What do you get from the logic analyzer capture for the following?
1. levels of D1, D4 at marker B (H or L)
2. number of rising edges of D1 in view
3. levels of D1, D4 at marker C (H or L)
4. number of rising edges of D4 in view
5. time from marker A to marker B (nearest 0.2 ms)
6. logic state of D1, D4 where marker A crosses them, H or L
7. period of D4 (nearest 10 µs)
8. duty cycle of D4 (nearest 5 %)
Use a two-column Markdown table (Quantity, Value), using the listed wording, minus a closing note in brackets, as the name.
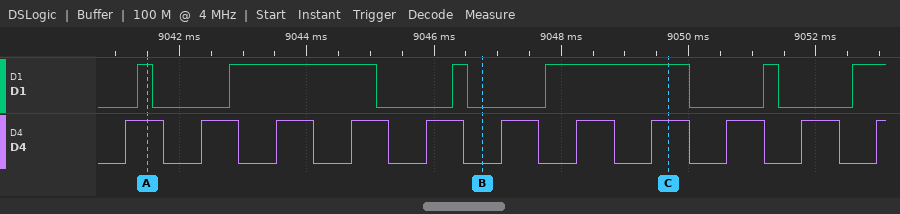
| Quantity | Value |
|---|---|
| levels of D1, D4 at marker B | D1=L, D4=L |
| number of rising edges of D1 in view | 6 |
| levels of D1, D4 at marker C | D1=H, D4=H |
| number of rising edges of D4 in view | 11 |
| time from marker A to marker B | 5.2 ms |
| logic state of D1, D4 where marker A crosses them, H or L | D1=H, D4=H |
| period of D4 | 1180 µs |
| duty cycle of D4 | 50 % |
